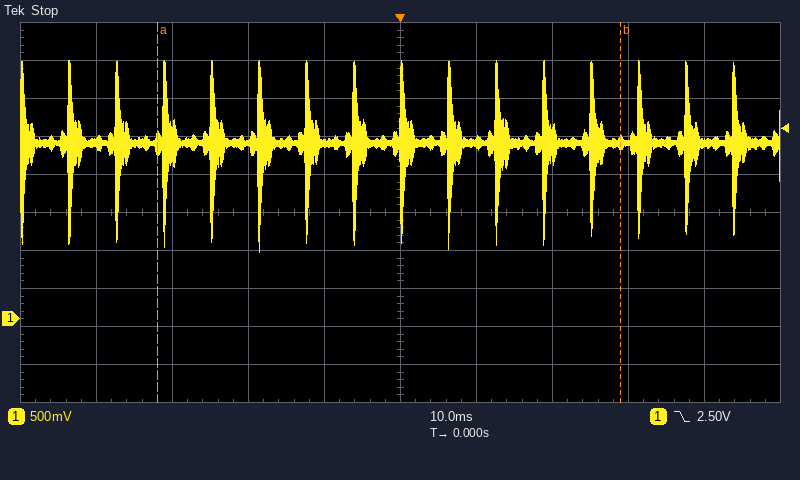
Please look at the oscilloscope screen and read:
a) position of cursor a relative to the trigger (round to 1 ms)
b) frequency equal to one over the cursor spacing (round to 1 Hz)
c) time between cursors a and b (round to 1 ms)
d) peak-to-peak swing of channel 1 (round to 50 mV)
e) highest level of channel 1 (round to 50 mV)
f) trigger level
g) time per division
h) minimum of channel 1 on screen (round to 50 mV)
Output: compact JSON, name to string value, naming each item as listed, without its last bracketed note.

{"position of cursor a relative to the trigger": "-32 ms", "frequency equal to one over the cursor spacing": "16 Hz", "time between cursors a and b": "61 ms", "peak-to-peak swing of channel 1": "2.50 V", "highest level of channel 1": "3.40 V", "trigger level": "2.50 V", "time per division": "10 ms", "minimum of channel 1 on screen": "900 mV"}
